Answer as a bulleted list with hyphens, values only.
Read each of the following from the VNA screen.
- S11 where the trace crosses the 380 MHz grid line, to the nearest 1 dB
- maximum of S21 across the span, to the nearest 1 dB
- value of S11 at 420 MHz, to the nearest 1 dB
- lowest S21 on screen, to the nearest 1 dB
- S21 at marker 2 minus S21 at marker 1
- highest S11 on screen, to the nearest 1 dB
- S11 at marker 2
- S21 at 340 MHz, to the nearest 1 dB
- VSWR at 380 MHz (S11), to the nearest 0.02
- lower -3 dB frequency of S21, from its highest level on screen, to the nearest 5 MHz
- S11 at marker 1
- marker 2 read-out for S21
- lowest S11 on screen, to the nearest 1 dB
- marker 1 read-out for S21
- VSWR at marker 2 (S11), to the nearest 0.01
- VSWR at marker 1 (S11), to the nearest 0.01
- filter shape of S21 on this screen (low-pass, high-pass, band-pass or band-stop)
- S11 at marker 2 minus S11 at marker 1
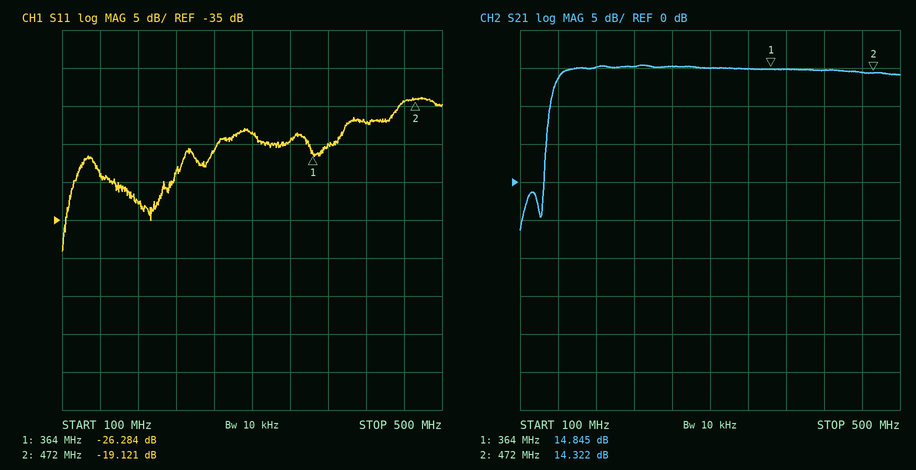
- -25 dB
- 15 dB
- -22 dB
- -6 dB
- -0.523 dB
- -19 dB
- -19.121 dB
- 15 dB
- 1.12
- 135 MHz
- -26.284 dB
- 14.322 dB
- -39 dB
- 14.845 dB
- 1.25
- 1.10
- high-pass
- 7.163 dB
